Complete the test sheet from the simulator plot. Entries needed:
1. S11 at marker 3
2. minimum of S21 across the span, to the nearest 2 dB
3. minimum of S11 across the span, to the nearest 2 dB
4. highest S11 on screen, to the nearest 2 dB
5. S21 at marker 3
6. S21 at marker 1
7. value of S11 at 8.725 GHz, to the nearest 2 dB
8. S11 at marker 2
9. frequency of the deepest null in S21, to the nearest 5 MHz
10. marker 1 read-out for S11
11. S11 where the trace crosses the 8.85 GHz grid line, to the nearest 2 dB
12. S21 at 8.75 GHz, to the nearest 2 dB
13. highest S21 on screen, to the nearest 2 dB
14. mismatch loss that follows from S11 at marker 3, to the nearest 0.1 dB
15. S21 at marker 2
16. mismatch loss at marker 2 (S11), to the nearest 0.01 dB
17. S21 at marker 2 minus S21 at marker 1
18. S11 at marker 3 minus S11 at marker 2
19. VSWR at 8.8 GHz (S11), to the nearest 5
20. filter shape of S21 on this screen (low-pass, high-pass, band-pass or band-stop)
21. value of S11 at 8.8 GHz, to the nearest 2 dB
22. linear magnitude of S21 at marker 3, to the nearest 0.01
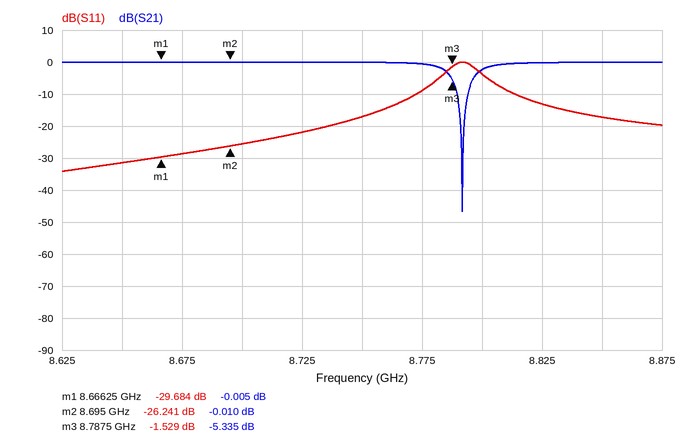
-1.529 dB
-46 dB
-34 dB
0 dB
-5.335 dB
-0.005 dB
-22 dB
-26.241 dB
8.790 GHz
-29.684 dB
-18 dB
0 dB
0 dB
5.3 dB
-0.010 dB
0.01 dB
-0.005 dB
24.712 dB
5
band-stop
-4 dB
0.54
